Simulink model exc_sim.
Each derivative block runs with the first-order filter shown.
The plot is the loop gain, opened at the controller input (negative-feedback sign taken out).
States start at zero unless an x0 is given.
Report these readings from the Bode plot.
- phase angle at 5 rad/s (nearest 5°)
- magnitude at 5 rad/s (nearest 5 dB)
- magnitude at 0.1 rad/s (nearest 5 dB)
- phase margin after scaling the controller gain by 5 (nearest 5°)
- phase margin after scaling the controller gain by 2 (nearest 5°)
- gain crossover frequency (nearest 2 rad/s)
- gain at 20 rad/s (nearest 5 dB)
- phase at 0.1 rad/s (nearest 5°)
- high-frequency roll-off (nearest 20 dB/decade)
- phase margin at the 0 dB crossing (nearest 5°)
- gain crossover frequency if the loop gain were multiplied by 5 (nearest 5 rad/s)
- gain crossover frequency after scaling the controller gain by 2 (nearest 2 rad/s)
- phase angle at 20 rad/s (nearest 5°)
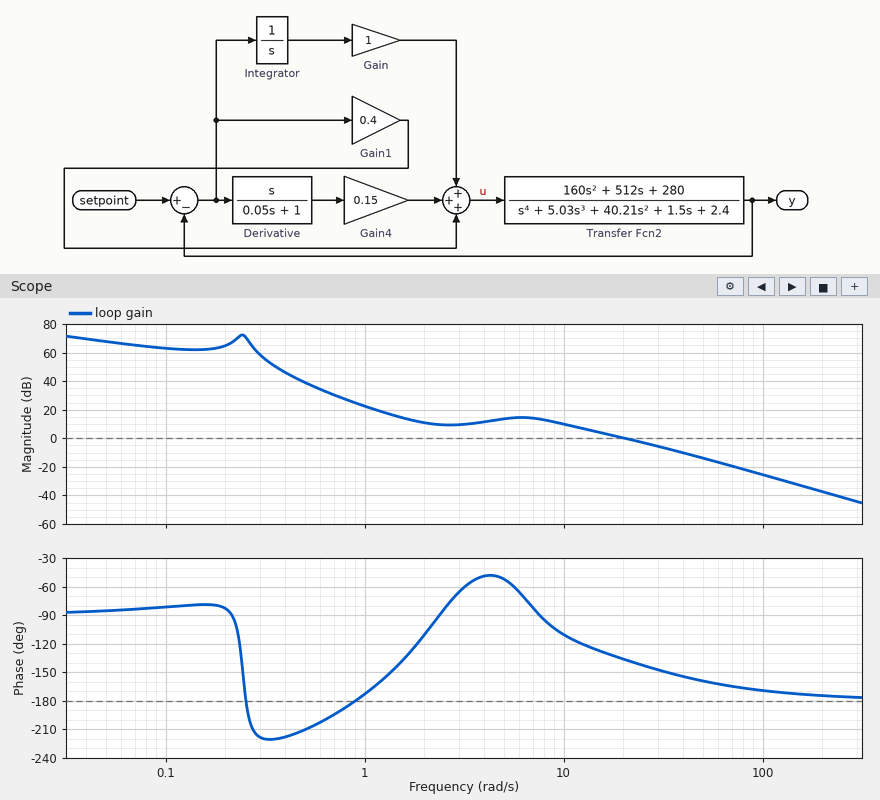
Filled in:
-50°
15 dB
65 dB
20°
30°
20 rad/s
0 dB
-80°
-40 dB/decade
45°
50 rad/s
30 rad/s
-135°
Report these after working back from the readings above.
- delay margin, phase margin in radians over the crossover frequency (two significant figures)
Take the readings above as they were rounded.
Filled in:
0.039 s
